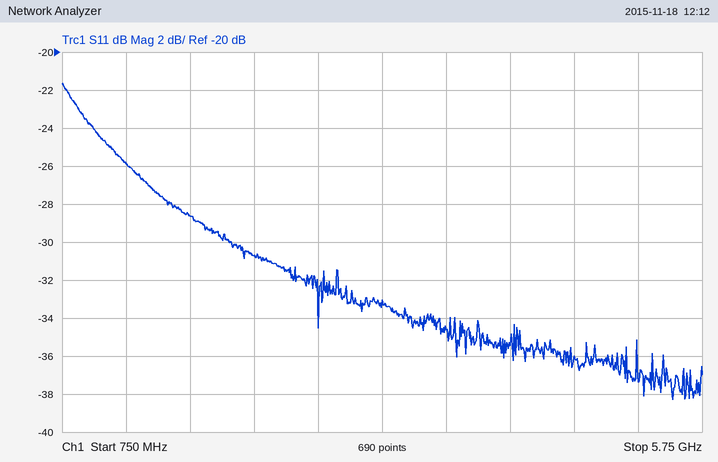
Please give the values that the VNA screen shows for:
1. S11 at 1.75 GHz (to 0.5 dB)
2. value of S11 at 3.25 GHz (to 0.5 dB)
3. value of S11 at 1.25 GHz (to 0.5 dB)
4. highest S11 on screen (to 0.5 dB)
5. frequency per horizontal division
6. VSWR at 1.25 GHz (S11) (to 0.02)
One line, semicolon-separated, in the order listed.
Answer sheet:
-28.5 dB; -33.0 dB; -26.0 dB; -21.5 dB; 500 MHz; 1.10
